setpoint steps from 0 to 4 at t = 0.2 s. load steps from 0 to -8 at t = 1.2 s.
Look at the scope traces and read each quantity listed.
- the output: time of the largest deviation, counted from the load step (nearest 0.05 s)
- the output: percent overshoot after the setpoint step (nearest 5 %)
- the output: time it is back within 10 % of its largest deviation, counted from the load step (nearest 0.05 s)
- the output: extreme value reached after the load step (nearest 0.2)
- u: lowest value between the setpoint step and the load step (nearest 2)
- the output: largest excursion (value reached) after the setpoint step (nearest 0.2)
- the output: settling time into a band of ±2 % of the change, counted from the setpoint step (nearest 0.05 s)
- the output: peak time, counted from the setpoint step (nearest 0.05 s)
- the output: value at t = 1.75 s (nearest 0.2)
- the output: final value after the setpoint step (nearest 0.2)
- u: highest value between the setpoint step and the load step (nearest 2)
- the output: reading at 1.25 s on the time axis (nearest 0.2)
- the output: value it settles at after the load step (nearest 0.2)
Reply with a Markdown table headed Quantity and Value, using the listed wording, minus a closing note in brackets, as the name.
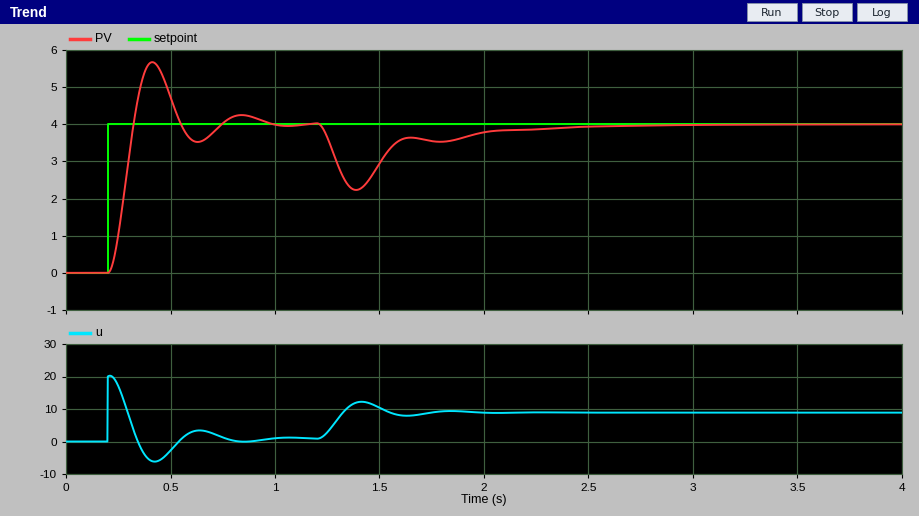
| Quantity | Value |
|---|---|
| the output: time of the largest deviation, counted from the load step | 0.20 s |
| the output: percent overshoot after the setpoint step | 40 % |
| the output: time it is back within 10 % of its largest deviation, counted from the load step | 0.85 s |
| the output: extreme value reached after the load step | 2.2 |
| u: lowest value between the setpoint step and the load step | -6 |
| the output: largest excursion (value reached) after the setpoint step | 5.6 |
| the output: settling time into a band of ±2 % of the change, counted from the setpoint step | 0.75 s |
| the output: peak time, counted from the setpoint step | 0.20 s |
| the output: value at t = 1.75 s | 3.6 |
| the output: final value after the setpoint step | 4.0 |
| u: highest value between the setpoint step and the load step | 20 |
| the output: reading at 1.25 s on the time axis | 3.6 |
| the output: value it settles at after the load step | 4.0 |
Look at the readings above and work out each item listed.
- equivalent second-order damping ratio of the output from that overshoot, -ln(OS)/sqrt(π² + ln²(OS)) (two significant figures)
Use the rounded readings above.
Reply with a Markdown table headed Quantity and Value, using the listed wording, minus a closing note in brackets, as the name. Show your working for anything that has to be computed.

| Quantity | Value |
|---|---|
| equivalent second-order damping ratio of the output from that overshoot, -ln(OS)/sqrt(π² + ln²(OS)) | ln(0.4) = -0.916; 0.916 / sqrt(9.870 + 0.840) = 0.28 |
